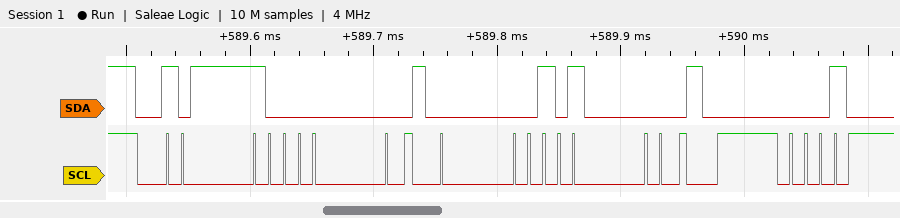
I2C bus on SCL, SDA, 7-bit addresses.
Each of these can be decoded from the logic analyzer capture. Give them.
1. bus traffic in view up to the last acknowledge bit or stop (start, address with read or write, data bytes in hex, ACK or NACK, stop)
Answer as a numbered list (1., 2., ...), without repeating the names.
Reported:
1. start, address 50 write ACK, 14 ACK
